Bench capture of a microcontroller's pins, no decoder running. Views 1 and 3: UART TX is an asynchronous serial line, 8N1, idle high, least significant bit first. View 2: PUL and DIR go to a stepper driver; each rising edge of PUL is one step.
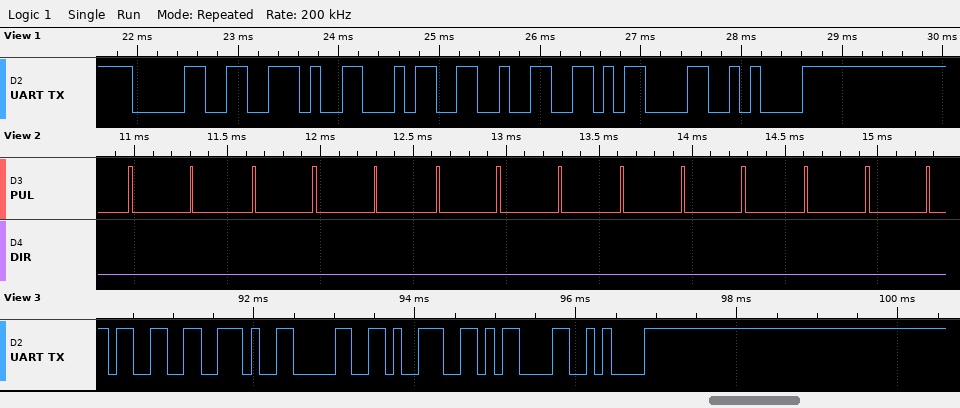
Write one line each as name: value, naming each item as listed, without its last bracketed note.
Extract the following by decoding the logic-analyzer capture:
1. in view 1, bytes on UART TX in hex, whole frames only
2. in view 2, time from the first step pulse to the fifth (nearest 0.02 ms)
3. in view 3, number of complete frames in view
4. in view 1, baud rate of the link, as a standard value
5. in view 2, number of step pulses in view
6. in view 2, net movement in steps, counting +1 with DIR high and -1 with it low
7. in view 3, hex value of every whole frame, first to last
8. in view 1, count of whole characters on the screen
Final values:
in view 1, bytes on UART TX in hex, whole frames only: 30 2E 34 32 0D 0A
in view 2, time from the first step pulse to the fifth: 1.32 ms
in view 3, number of complete frames in view: 6
in view 1, baud rate of the link, as a standard value: 9600 baud
in view 2, number of step pulses in view: 14
in view 2, net movement in steps, counting +1 with DIR high and -1 with it low: -14
in view 3, hex value of every whole frame, first to last: 33 2E 30 39 0D 0A
in view 1, count of whole characters on the screen: 6
